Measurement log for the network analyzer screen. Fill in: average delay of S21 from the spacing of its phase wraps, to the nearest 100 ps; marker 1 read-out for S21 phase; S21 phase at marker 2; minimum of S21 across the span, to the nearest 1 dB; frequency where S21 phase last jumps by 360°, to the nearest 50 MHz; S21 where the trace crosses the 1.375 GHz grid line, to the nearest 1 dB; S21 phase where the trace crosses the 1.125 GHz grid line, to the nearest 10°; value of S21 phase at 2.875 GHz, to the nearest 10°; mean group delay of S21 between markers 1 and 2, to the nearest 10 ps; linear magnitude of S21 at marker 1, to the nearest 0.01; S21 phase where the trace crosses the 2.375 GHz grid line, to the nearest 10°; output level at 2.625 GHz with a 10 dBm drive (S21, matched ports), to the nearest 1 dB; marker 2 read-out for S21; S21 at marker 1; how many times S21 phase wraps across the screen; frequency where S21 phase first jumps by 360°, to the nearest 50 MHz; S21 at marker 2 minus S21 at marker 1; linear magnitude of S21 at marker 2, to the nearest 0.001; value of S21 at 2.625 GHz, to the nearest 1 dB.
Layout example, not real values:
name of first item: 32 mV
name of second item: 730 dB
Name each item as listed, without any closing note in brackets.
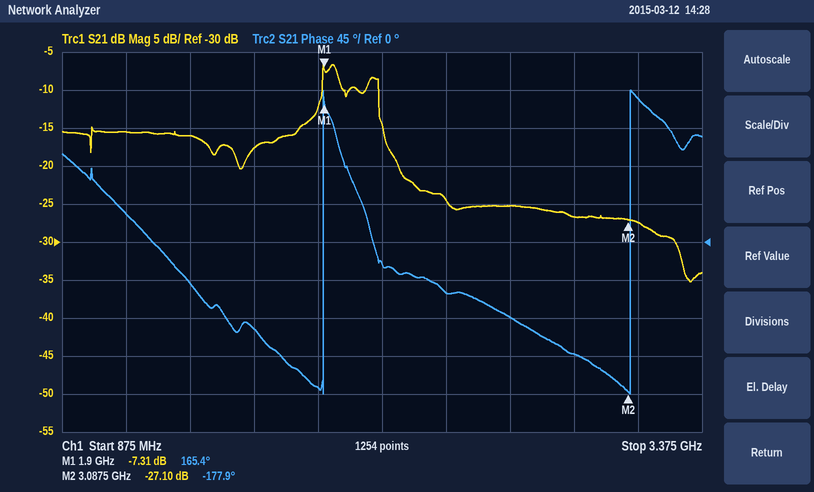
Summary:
average delay of S21 from the spacing of its phase wraps, to the nearest 100 ps: 800 ps
marker 1 read-out for S21 phase: 165.4°
S21 phase at marker 2: -177.9°
minimum of S21 across the span, to the nearest 1 dB: -35 dB
frequency where S21 phase last jumps by 360°, to the nearest 50 MHz: 3.10 GHz
S21 where the trace crosses the 1.375 GHz grid line, to the nearest 1 dB: -16 dB
S21 phase where the trace crosses the 1.125 GHz grid line, to the nearest 10°: 30°
value of S21 phase at 2.875 GHz, to the nearest 10°: -130°
mean group delay of S21 between markers 1 and 2, to the nearest 10 ps: 800 ps
linear magnitude of S21 at marker 1, to the nearest 0.01: 0.43
S21 phase where the trace crosses the 2.375 GHz grid line, to the nearest 10°: -60°
output level at 2.625 GHz with a 10 dBm drive (S21, matched ports), to the nearest 1 dB: -15 dBm
marker 2 read-out for S21: -27.10 dB
S21 at marker 1: -7.31 dB
how many times S21 phase wraps across the screen: 2
frequency where S21 phase first jumps by 360°, to the nearest 50 MHz: 1.90 GHz
S21 at marker 2 minus S21 at marker 1: -19.79 dB
linear magnitude of S21 at marker 2, to the nearest 0.001: 0.044
value of S21 at 2.625 GHz, to the nearest 1 dB: -25 dB
